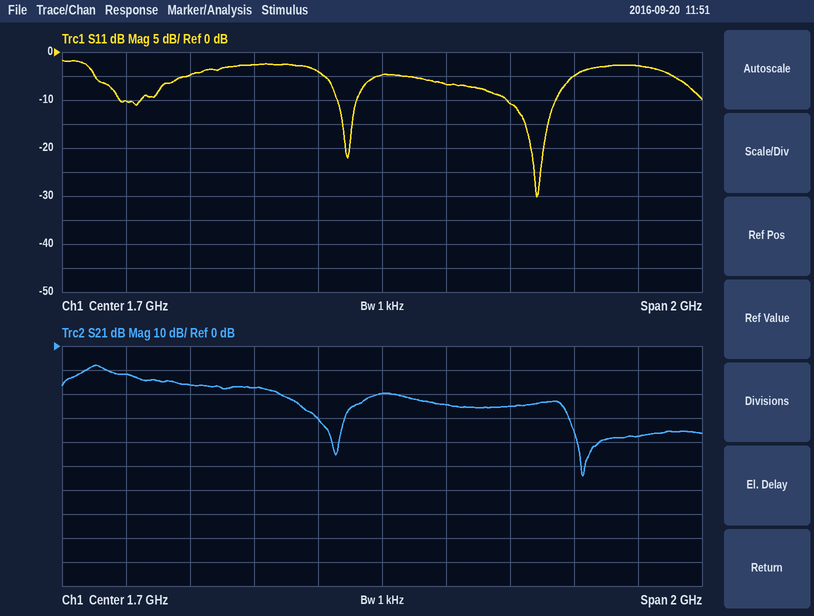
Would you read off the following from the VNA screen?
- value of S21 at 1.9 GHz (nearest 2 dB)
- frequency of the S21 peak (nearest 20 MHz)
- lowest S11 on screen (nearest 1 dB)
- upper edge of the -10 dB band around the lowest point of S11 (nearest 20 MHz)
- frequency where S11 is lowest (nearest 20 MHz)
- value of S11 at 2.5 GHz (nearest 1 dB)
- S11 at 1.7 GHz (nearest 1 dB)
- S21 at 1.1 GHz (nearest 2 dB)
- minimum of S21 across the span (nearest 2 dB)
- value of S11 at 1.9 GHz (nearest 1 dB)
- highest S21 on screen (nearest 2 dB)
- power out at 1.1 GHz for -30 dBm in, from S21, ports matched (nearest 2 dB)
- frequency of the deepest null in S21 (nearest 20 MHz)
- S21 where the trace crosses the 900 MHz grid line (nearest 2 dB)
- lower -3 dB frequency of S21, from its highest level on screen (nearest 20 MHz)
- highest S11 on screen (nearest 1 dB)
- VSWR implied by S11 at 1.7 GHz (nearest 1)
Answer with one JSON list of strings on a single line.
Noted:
["-24 dB", "800 MHz", "-30 dB", "2.24 GHz", "2.18 GHz", "-3 dB", "-5 dB", "-16 dB", "-54 dB", "-7 dB", "-8 dB", "-46 dBm", "2.32 GHz", "-12 dB", "760 MHz", "-2 dB", "4"]
